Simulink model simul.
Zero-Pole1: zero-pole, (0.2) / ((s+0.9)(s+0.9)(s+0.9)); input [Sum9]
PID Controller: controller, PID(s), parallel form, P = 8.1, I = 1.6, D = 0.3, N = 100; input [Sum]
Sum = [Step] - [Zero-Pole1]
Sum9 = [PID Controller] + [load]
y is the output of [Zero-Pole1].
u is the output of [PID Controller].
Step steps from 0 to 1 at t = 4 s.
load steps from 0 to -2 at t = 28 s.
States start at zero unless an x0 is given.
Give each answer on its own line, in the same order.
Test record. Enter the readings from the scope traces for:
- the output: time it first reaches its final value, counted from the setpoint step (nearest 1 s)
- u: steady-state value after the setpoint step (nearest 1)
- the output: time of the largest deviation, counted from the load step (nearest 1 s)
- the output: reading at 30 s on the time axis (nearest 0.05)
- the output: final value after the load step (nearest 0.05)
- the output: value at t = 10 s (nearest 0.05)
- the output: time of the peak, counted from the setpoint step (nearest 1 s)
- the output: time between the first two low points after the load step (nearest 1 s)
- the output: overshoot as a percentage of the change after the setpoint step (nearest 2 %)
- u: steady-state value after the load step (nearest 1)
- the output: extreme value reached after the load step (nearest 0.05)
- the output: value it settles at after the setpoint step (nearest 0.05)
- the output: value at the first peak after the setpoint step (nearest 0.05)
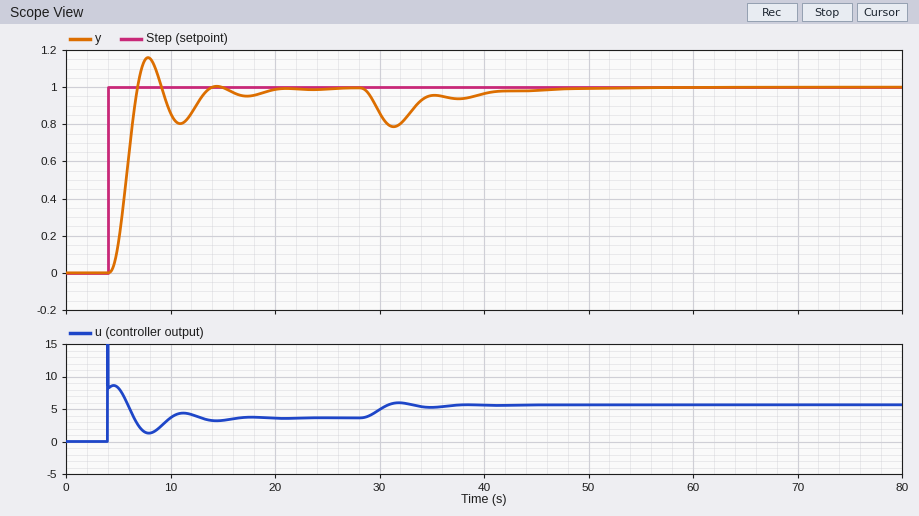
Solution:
3 s
4
3 s
0.85
1.00
0.85
4 s
6 s
16 %
6
0.80
1.00
1.15
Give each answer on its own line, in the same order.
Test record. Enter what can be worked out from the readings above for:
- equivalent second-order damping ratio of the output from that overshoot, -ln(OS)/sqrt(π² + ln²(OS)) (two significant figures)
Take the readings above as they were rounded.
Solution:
0.50
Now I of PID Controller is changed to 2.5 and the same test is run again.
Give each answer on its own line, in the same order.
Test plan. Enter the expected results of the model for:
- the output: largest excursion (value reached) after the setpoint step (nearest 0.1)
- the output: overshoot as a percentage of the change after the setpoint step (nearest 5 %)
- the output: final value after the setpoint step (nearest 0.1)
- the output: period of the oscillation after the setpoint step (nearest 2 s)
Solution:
1.3
30 %
1.0
6 s
